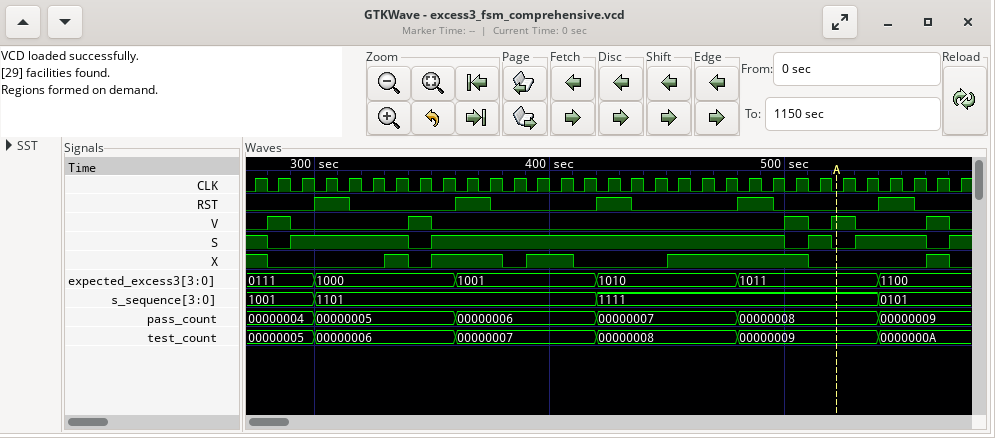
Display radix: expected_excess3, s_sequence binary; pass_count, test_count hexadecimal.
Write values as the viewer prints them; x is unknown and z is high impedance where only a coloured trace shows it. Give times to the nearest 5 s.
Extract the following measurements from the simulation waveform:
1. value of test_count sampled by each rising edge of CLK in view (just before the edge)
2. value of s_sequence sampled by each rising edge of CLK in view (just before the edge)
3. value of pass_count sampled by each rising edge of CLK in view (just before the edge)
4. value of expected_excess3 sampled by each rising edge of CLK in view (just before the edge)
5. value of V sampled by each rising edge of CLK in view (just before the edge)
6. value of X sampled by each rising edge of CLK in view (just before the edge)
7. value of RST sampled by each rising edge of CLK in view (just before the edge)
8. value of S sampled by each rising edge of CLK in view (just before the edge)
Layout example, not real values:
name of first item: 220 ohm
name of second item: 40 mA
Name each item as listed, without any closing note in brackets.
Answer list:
value of test_count sampled by each rising edge of CLK in view: 00000005, 00000005, 00000005, 00000006, 00000006, 00000006, 00000006, 00000006, 00000006, 00000007, 00000007, 00000007, 00000007, 00000007, 00000007, 00000008, 00000008, 00000008, 00000008, 00000008, 00000008, 00000009, 00000009, 00000009, 00000009, 00000009, 00000009, 0000000A, 0000000A, 0000000A, 0000000A
value of s_sequence sampled by each rising edge of CLK in view: 1001, 1001, 1001, 1101, 1101, 1101, 1101, 1101, 1101, 1101, 1101, 1101, 1101, 1101, 1101, 1111, 1111, 1111, 1111, 1111, 1111, 1111, 1111, 1111, 1111, 1111, 1111, 0101, 0101, 0101, 0101
value of pass_count sampled by each rising edge of CLK in view: 00000004, 00000004, 00000004, 00000005, 00000005, 00000005, 00000005, 00000005, 00000005, 00000006, 00000006, 00000006, 00000006, 00000006, 00000006, 00000007, 00000007, 00000007, 00000007, 00000007, 00000007, 00000008, 00000008, 00000008, 00000008, 00000008, 00000008, 00000009, 00000009, 00000009, 00000009
value of expected_excess3 sampled by each rising edge of CLK in view: 0111, 0111, 0111, 1000, 1000, 1000, 1000, 1000, 1000, 1001, 1001, 1001, 1001, 1001, 1001, 1010, 1010, 1010, 1010, 1010, 1010, 1011, 1011, 1011, 1011, 1011, 1011, 1100, 1100, 1100, 1100
value of V sampled by each rising edge of CLK in view: 0 1 0 0 0 0 0 1 0 0 0 0 0 0 0 0 0 0 0 0 0 0 0 1 0 1 0 0 0 1 0
value of X sampled by each rising edge of CLK in view: 1 0 0 0 0 0 1 0 1 1 1 0 1 1 0 0 0 0 1 1 1 1 1 1 0 0 0 0 0 1 0
value of RST sampled by each rising edge of CLK in view: 0 0 0 1 1 0 0 0 0 1 1 0 0 0 0 1 1 0 0 0 0 1 1 0 0 0 0 1 1 0 0
value of S sampled by each rising edge of CLK in view: 1 0 1 1 1 1 1 0 1 1 1 1 1 1 1 1 1 1 1 1 1 1 1 0 1 0 1 1 1 0 1
